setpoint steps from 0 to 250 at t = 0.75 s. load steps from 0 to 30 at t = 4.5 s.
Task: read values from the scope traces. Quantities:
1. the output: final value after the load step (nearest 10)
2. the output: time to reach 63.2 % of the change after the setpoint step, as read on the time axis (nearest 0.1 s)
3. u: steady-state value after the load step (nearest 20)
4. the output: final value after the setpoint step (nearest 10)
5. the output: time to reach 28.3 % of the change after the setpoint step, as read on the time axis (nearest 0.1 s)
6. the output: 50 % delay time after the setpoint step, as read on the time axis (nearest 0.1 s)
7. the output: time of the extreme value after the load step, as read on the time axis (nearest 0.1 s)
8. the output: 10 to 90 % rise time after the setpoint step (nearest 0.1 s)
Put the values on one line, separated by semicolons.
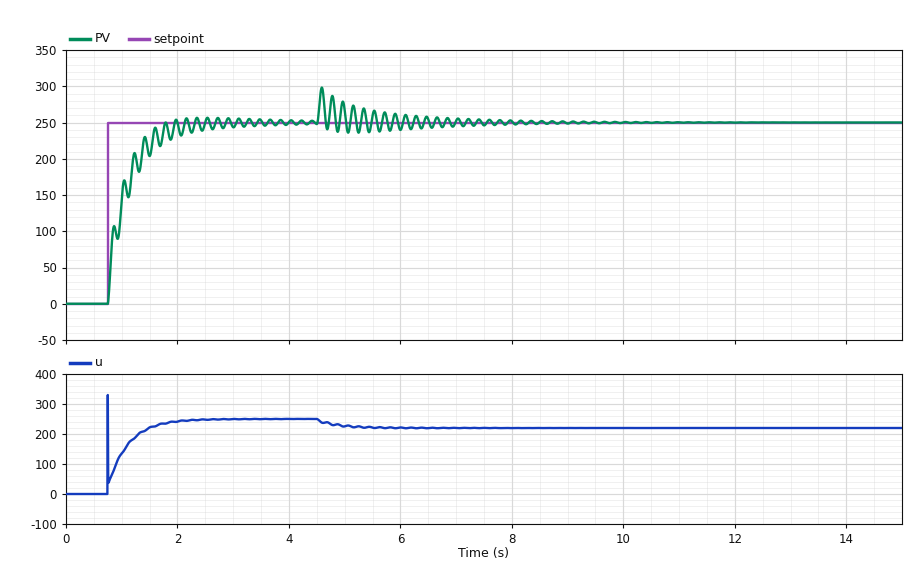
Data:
250; 1.0 s; 220; 250; 0.8 s; 1.0 s; 4.6 s; 0.6 s
